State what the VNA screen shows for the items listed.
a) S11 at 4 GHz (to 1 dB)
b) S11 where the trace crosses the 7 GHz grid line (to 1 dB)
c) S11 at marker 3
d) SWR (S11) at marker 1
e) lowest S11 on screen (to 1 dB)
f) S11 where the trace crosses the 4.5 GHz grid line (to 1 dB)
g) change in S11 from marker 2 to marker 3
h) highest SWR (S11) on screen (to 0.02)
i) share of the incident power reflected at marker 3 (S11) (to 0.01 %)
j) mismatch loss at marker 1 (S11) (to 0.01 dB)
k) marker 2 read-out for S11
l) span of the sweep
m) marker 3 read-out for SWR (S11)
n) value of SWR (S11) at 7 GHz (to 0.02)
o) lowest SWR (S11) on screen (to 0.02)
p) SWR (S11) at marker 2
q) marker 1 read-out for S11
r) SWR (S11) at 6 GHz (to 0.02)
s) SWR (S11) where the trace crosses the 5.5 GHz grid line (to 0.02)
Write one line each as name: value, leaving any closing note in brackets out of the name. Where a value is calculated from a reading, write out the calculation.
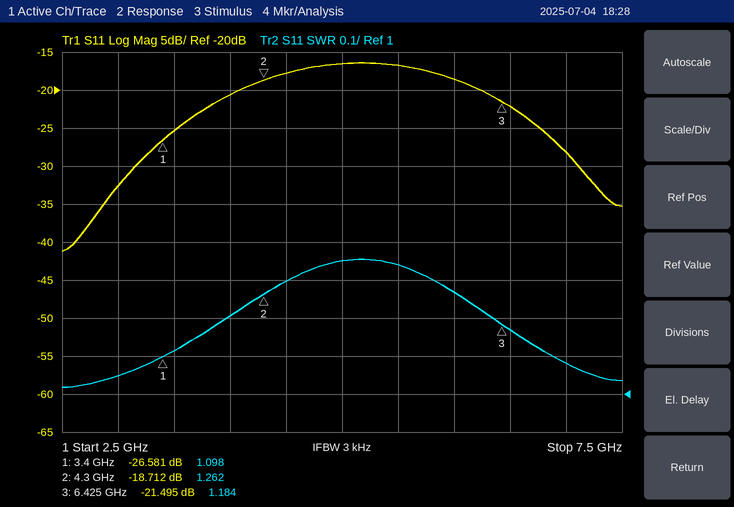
S11 at 4 GHz: -21 dB
S11 where the trace crosses the 7 GHz grid line: -28 dB
S11 at marker 3: -21.495 dB
SWR (S11) at marker 1: 1.098
lowest S11 on screen: -41 dB
S11 where the trace crosses the 4.5 GHz grid line: -18 dB
change in S11 from marker 2 to marker 3: -21.495 − (-18.712) = -2.783 dB
highest SWR (S11) on screen: 1.36
share of the incident power reflected at marker 3 (S11): 10^(-21.495/10) ≈ 0.71 %
mismatch loss at marker 1 (S11): −10 log10(1 − 10^(-26.581/10)) ≈ 0.01 dB
marker 2 read-out for S11: -18.712 dB
span of the sweep: 5 GHz
marker 3 read-out for SWR: 1.184
value of SWR (S11) at 7 GHz: 1.08
lowest SWR (S11) on screen: 1.02
SWR (S11) at marker 2: 1.262
marker 1 read-out for S11: -26.581 dB
SWR (S11) at 6 GHz: 1.26
SWR (S11) where the trace crosses the 5.5 GHz grid line: 1.34
